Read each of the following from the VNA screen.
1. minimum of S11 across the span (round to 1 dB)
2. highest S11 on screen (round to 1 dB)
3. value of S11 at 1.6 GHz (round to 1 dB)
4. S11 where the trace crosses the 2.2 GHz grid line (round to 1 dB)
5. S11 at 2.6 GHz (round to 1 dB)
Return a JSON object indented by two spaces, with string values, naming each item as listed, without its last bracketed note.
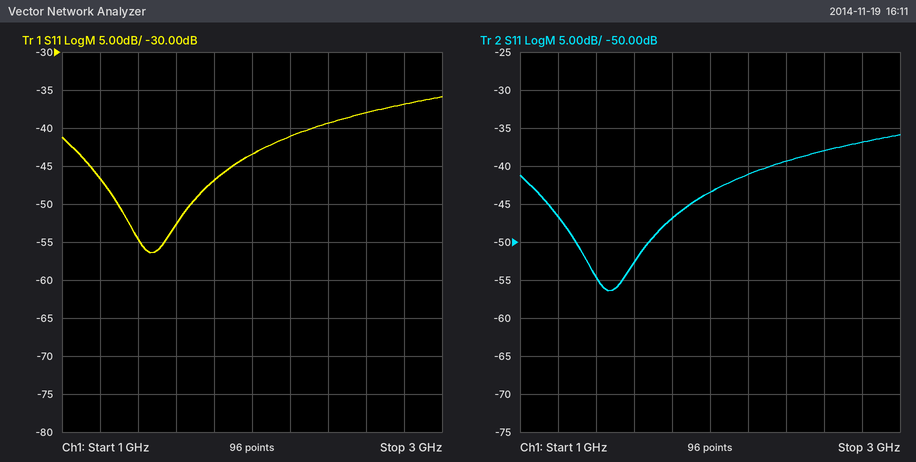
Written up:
{
  "minimum of S11 across the span": "-56 dB",
  "highest S11 on screen": "-36 dB",
  "value of S11 at 1.6 GHz": "-53 dB",
  "S11 where the trace crosses the 2.2 GHz grid line": "-41 dB",
  "S11 at 2.6 GHz": "-38 dB"
}
